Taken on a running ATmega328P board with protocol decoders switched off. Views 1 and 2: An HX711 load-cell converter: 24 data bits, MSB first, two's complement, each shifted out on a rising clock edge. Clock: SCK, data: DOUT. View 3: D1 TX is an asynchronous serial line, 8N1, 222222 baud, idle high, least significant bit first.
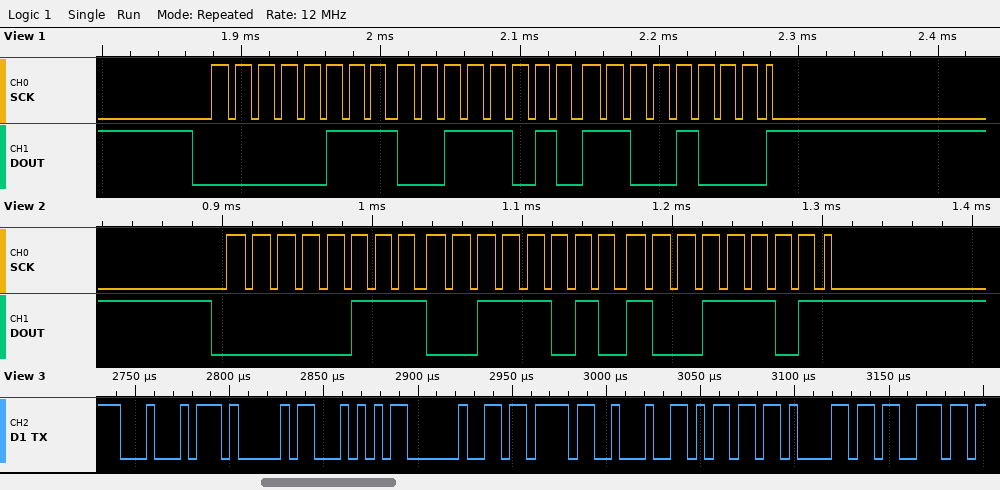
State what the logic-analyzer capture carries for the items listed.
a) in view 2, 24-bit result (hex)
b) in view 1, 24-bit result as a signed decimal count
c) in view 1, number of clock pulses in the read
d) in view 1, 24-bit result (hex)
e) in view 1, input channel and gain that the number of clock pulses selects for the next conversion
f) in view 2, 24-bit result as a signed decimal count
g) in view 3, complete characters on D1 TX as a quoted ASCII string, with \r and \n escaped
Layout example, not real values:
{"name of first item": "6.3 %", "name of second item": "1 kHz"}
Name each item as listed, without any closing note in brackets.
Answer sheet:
{"in view 2, 24-bit result": "0x073A9D", "in view 1, 24-bit result as a signed decimal count": "473800", "in view 1, number of clock pulses in the read": "25", "in view 1, 24-bit result": "0x073AC8", "in view 1, input channel and gain that the number of clock pulses selects for the next conversion": "channel A, gain 128", "in view 2, 24-bit result as a signed decimal count": "473757", "in view 3, complete characters on D1 TX as a quoted ASCII string, with \\r and \\n escaped": "\"DAT {\\\"mas\""}
